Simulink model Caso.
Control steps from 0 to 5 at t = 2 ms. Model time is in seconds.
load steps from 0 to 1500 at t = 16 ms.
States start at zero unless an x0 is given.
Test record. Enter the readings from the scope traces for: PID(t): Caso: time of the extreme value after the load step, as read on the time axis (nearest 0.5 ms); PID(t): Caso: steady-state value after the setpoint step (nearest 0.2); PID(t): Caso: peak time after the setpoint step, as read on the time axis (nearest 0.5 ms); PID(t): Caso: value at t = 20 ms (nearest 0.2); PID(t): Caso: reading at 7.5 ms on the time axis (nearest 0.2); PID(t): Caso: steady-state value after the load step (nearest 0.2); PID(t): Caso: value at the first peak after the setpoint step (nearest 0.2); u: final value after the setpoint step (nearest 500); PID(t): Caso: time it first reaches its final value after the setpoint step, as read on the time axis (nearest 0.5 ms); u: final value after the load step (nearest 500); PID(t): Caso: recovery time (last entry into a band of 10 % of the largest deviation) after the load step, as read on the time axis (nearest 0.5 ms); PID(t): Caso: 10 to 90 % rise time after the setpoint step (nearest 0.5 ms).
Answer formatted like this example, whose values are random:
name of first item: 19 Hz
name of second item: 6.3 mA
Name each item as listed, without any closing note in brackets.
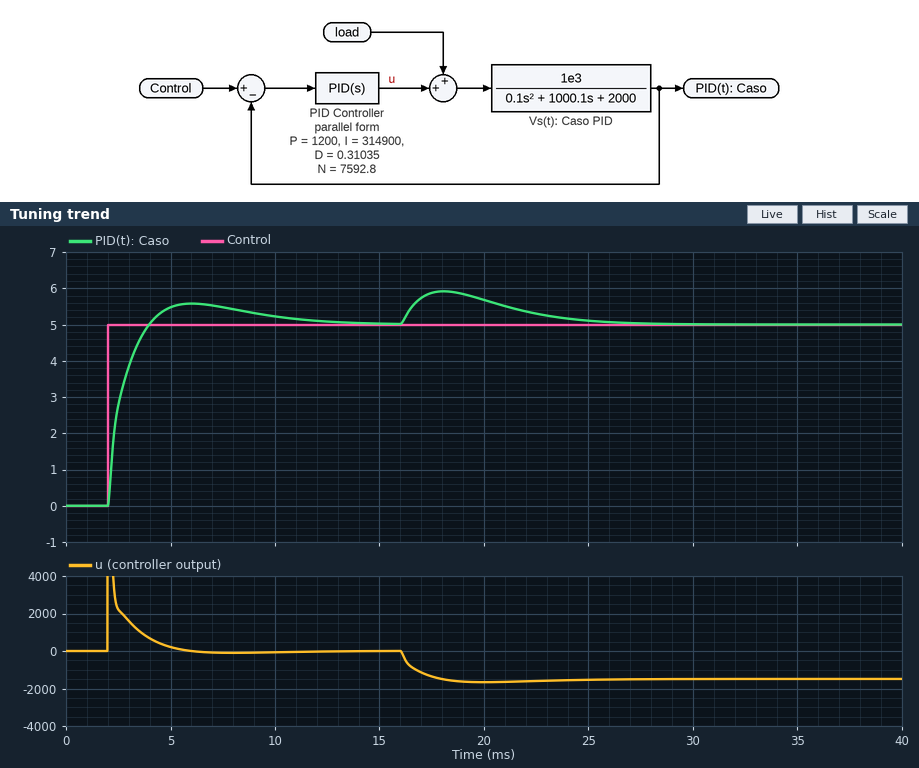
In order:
PID(t): Caso: time of the extreme value after the load step, as read on the time axis: 18.0 ms
PID(t): Caso: steady-state value after the setpoint step: 5.0
PID(t): Caso: peak time after the setpoint step, as read on the time axis: 6.0 ms
PID(t): Caso: value at t = 20 ms: 5.6
PID(t): Caso: reading at 7.5 ms on the time axis: 5.4
PID(t): Caso: steady-state value after the load step: 5.0
PID(t): Caso: value at the first peak after the setpoint step: 5.6
u: final value after the setpoint step: 0
PID(t): Caso: time it first reaches its final value after the setpoint step, as read on the time axis: 4.0 ms
u: final value after the load step: -1500
PID(t): Caso: recovery time (last entry into a band of 10 % of the largest deviation) after the load step, as read on the time axis: 25.5 ms
PID(t): Caso: 10 to 90 % rise time after the setpoint step: 1.5 ms
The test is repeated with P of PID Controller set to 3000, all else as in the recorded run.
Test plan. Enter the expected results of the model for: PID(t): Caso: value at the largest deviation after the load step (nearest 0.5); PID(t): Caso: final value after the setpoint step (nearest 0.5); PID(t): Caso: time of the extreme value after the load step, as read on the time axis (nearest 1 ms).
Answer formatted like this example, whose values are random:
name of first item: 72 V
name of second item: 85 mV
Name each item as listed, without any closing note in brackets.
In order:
PID(t): Caso: value at the largest deviation after the load step: 5.5
PID(t): Caso: final value after the setpoint step: 5.0
PID(t): Caso: time of the extreme value after the load step, as read on the time axis: 17 ms
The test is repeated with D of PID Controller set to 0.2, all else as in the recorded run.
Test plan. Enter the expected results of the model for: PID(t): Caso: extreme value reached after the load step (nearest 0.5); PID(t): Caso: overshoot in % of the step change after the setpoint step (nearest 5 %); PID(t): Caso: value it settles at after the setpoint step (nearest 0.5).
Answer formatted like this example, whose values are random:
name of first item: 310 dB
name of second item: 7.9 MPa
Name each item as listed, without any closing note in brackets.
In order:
PID(t): Caso: extreme value reached after the load step: 6.0
PID(t): Caso: overshoot in % of the step change after the setpoint step: 10 %
PID(t): Caso: value it settles at after the setpoint step: 5.0
